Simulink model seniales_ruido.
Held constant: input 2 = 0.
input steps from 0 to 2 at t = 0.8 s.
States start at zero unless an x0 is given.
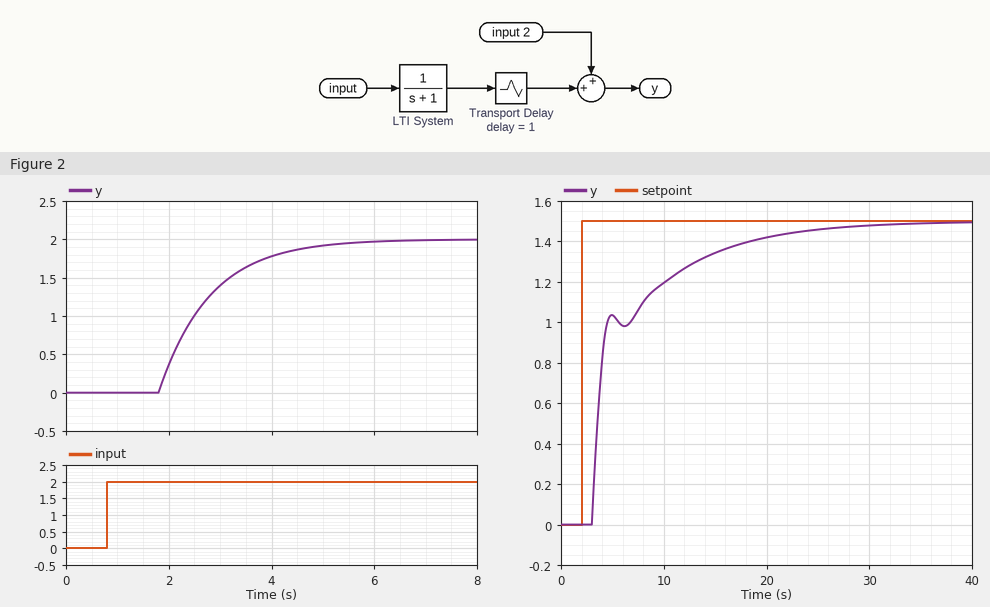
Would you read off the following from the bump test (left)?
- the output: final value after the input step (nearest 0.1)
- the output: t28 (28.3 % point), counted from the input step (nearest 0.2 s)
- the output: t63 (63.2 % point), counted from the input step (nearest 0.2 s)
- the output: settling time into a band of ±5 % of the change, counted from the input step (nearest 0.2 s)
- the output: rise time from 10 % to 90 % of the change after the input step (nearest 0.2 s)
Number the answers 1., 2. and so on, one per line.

1. 2.0
2. 1.4 s
3. 2.0 s
4. 4.0 s
5. 2.2 s
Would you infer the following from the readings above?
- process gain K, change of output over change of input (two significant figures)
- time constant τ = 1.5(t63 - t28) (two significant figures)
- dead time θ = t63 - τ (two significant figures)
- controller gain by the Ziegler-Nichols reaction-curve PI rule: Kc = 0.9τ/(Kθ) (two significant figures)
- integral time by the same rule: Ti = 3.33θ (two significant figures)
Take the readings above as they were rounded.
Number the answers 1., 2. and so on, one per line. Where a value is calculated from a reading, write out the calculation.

1. (2 - 0) / 2 = 1.0
2. 1.5 × (2 - 1.4) = 0.90 s
3. 2 - 0.9 = 1.1 s
4. 0.9 × 0.9 / (1 × 1.1) = 0.74
5. 3.33 × 1.1 = 3.7 s
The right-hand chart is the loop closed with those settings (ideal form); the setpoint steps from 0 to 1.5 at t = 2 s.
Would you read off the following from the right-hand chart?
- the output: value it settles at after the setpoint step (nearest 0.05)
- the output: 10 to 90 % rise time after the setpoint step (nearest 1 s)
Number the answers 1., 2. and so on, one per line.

1. 1.50
2. 12 s
